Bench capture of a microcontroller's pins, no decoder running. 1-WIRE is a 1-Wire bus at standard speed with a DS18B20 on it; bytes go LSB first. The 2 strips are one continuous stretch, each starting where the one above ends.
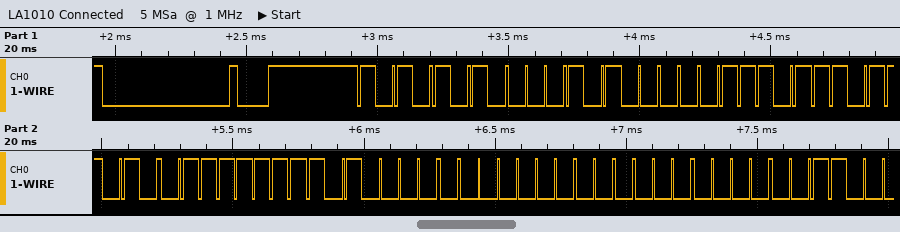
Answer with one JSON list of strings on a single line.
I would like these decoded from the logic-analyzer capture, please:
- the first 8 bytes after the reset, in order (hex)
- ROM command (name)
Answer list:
["55 28 B8 5B FE 05 00 00", "Match ROM"]
